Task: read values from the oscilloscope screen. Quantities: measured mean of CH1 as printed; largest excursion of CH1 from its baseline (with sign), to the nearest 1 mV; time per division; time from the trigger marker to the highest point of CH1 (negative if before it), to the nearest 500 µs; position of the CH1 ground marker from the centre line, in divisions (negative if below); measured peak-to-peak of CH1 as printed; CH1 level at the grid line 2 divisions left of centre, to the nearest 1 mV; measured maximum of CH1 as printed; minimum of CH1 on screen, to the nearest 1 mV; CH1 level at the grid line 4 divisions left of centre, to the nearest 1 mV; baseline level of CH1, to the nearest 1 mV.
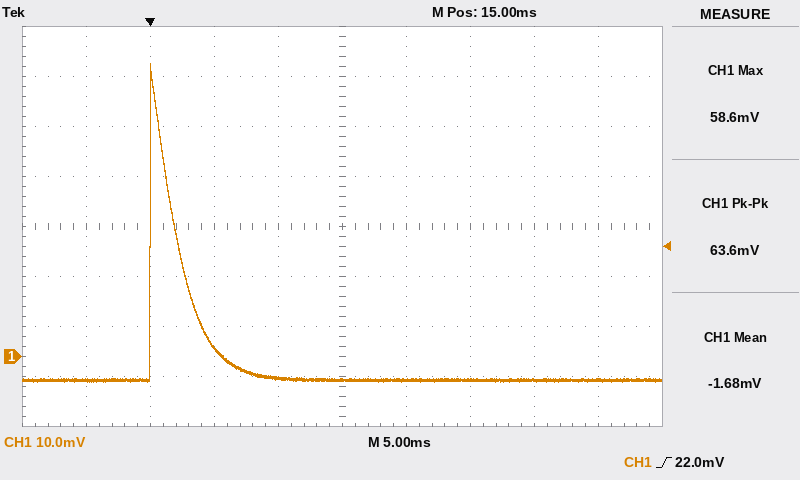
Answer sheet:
-1.68 mV
+63 mV
5 ms
0.0 ms
-2.6 div
63.6 mV
2 mV
58.6 mV
-5 mV
-5 mV
-5 mV
